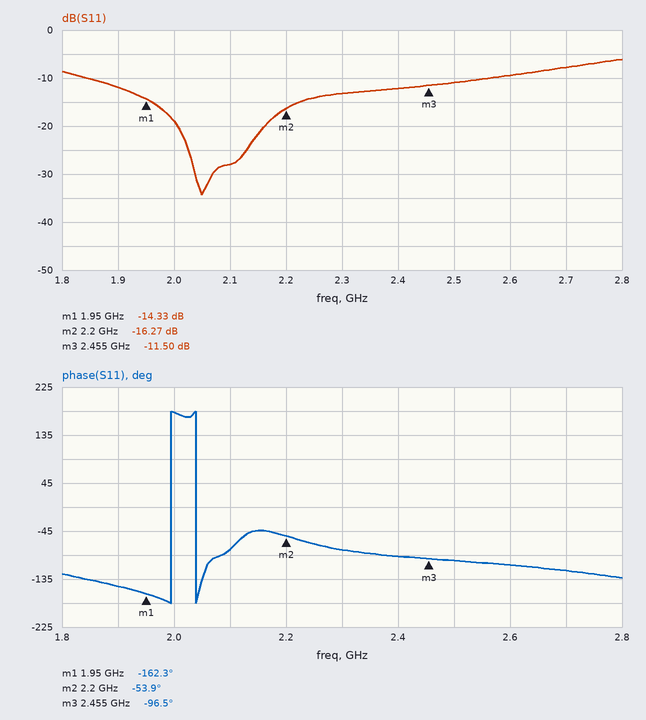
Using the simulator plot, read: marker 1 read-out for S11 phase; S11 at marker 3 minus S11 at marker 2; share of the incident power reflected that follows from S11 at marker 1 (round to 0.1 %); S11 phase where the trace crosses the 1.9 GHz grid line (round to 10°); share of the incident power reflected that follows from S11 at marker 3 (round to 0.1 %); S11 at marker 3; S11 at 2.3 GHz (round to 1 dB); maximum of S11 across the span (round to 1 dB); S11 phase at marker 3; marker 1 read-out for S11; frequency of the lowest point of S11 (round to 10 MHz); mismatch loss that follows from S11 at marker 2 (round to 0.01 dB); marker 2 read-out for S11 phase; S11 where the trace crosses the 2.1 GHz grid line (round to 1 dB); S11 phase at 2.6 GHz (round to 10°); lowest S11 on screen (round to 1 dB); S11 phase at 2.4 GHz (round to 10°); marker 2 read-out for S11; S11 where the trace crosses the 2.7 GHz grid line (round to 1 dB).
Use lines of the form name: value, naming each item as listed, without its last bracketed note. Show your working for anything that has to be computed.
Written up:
marker 1 read-out for S11 phase: -162.3°
S11 at marker 3 minus S11 at marker 2: -11.5 − (-16.27) = 4.77 dB
share of the incident power reflected that follows from S11 at marker 1: 10^(-14.33/10) ≈ 3.7 %
S11 phase where the trace crosses the 1.9 GHz grid line: -150°
share of the incident power reflected that follows from S11 at marker 3: 10^(-11.5/10) ≈ 7.1 %
S11 at marker 3: -11.50 dB
S11 at 2.3 GHz: -13 dB
maximum of S11 across the span: -6 dB
S11 phase at marker 3: -96.5°
marker 1 read-out for S11: -14.33 dB
frequency of the lowest point of S11: 2.05 GHz
mismatch loss that follows from S11 at marker 2: −10 log10(1 − 10^(-16.27/10)) ≈ 0.10 dB
marker 2 read-out for S11 phase: -53.9°
S11 where the trace crosses the 2.1 GHz grid line: -28 dB
S11 phase at 2.6 GHz: -110°
lowest S11 on screen: -34 dB
S11 phase at 2.4 GHz: -90°
marker 2 read-out for S11: -16.27 dB
S11 where the trace crosses the 2.7 GHz grid line: -8 dB
